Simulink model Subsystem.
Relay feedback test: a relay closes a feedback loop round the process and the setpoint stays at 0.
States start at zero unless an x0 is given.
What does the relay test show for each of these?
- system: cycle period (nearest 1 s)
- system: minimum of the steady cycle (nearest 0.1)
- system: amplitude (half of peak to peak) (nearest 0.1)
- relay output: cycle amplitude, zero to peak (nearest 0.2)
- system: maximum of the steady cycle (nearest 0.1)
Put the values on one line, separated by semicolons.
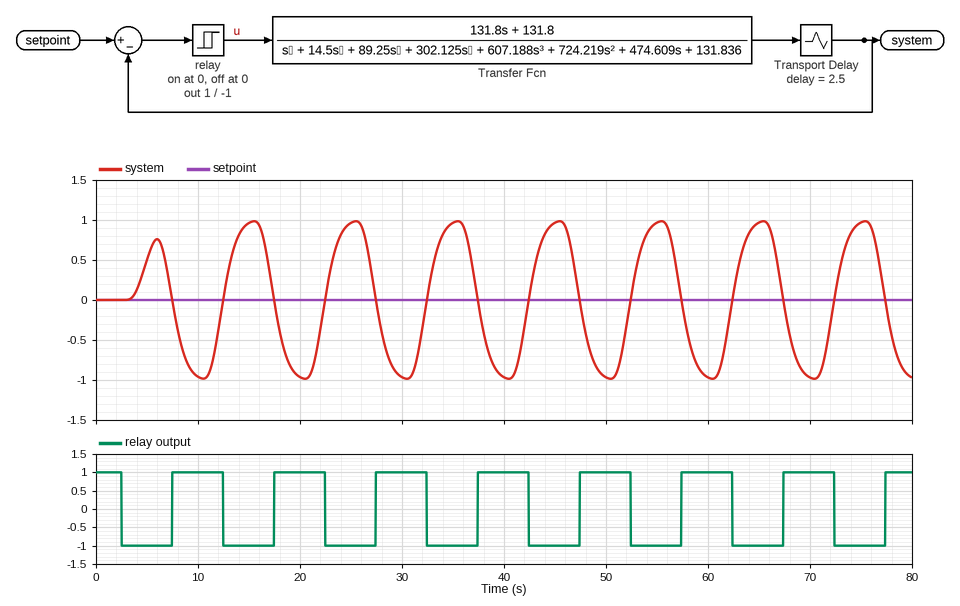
10 s; -1.0; 1.0; 1.0; 1.0
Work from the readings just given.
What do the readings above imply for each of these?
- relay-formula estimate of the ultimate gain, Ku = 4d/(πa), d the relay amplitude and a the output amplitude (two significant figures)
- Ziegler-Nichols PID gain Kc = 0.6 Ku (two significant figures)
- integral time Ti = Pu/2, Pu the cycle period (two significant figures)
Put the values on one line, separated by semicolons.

1.3; 0.78; 5.0 s
